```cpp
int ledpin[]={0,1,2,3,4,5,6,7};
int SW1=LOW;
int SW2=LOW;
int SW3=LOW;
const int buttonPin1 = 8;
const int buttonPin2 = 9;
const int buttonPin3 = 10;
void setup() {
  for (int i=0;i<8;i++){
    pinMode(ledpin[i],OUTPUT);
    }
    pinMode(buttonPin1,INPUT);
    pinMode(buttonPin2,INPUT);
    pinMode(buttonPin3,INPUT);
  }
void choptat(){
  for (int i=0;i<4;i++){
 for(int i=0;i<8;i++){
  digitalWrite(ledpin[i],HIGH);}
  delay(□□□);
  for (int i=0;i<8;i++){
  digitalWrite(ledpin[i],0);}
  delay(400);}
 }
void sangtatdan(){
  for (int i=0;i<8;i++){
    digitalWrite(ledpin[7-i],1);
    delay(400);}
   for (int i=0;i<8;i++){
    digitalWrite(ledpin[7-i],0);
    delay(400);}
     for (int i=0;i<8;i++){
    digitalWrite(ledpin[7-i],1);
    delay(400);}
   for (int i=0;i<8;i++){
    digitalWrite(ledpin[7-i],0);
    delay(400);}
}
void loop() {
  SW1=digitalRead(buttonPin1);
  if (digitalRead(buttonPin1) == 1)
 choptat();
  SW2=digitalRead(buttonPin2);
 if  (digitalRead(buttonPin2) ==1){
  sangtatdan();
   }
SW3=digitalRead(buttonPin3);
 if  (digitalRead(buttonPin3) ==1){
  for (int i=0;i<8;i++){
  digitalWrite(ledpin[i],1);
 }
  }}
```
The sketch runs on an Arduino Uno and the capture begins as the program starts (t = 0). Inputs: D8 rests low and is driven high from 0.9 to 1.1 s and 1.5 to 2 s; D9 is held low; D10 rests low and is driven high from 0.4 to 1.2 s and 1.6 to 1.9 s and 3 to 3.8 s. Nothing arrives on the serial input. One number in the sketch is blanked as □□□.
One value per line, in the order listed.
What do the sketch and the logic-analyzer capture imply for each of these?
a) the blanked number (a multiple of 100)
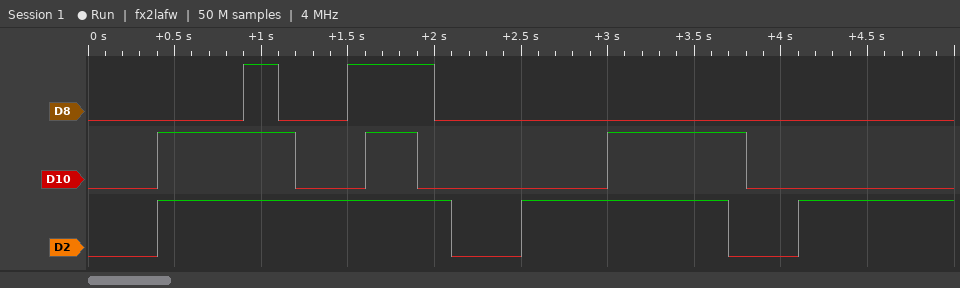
1200
